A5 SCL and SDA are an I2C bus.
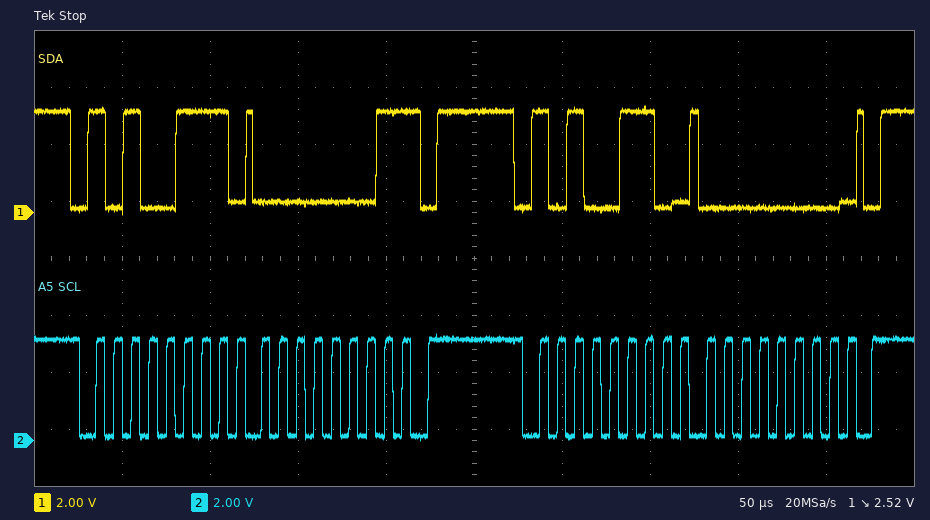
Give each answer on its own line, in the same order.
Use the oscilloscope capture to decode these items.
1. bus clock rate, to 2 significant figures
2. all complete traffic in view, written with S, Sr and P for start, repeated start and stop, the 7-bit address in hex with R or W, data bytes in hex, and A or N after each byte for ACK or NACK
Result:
100 kHz
S 53R A 01 N P S 53W A 00 A P
